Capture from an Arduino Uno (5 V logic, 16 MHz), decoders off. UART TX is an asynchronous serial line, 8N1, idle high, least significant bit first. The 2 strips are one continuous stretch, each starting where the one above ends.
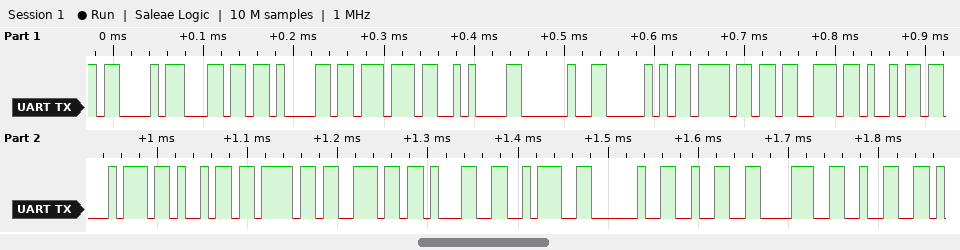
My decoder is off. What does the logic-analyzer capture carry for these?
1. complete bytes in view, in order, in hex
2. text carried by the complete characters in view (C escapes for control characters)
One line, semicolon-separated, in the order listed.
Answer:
43 6C 61 77 0A 20 50 6F 73 69 74 69 6F 6E 31 3A 20 32 38 32; "Claw\n Position1: 282"
